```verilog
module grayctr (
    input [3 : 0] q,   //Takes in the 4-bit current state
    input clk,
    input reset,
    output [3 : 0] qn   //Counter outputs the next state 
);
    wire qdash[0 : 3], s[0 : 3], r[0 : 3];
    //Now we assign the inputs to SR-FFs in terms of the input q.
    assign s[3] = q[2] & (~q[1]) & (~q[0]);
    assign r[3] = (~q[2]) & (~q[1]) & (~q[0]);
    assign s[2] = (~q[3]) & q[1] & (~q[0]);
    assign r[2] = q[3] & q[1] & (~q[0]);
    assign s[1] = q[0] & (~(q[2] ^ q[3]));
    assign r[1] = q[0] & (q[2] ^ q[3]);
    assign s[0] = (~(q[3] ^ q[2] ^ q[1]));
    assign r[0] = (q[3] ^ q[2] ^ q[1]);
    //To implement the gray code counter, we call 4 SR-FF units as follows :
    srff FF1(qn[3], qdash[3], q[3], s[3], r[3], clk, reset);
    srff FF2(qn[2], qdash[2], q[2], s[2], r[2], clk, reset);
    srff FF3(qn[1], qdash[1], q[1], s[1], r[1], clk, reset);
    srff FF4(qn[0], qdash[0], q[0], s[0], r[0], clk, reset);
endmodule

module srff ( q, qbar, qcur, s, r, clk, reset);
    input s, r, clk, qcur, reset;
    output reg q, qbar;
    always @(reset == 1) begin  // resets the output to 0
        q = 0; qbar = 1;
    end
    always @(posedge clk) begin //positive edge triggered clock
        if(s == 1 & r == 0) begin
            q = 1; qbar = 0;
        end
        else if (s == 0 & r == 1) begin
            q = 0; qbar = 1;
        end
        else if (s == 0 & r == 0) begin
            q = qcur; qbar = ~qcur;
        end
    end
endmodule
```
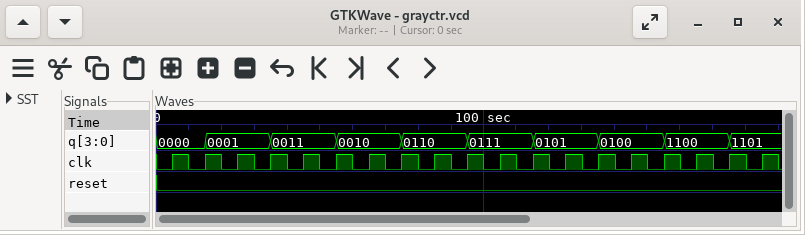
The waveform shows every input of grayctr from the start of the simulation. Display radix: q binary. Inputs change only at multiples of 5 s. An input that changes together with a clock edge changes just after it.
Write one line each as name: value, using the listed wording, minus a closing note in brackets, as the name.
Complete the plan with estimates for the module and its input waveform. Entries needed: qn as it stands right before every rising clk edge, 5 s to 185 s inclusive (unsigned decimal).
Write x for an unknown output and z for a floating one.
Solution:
qn as it stands right before every rising clk edge, 5 s to 185 s inclusive: 0, 1, 1, 3, 3, 2, 2, 6, 6, 7, 7, 5, 5, 4, 4, 12, 12, 13, 13
